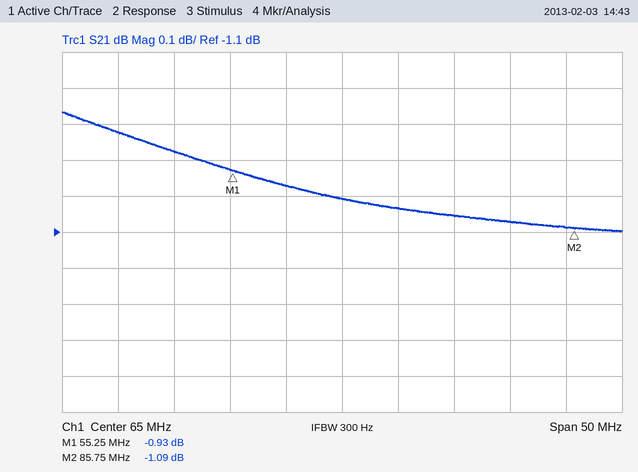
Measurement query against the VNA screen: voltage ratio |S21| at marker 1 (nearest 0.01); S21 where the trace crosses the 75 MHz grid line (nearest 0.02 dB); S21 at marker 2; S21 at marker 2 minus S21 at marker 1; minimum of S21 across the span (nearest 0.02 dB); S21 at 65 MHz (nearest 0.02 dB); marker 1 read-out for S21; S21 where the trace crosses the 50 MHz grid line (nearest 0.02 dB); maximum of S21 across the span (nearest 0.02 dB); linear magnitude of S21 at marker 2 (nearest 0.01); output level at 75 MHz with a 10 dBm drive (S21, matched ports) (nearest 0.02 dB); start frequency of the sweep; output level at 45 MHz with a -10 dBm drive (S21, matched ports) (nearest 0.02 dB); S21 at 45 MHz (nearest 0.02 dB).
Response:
0.90
-1.06 dB
-1.09 dB
-0.16 dB
-1.10 dB
-1.00 dB
-0.93 dB
-0.88 dB
-0.76 dB
0.88
8.94 dBm
40 MHz
-10.82 dBm
-0.82 dB
